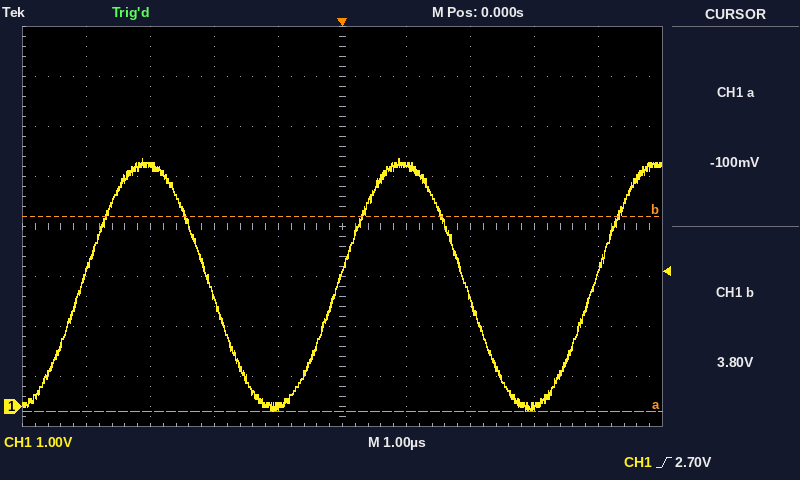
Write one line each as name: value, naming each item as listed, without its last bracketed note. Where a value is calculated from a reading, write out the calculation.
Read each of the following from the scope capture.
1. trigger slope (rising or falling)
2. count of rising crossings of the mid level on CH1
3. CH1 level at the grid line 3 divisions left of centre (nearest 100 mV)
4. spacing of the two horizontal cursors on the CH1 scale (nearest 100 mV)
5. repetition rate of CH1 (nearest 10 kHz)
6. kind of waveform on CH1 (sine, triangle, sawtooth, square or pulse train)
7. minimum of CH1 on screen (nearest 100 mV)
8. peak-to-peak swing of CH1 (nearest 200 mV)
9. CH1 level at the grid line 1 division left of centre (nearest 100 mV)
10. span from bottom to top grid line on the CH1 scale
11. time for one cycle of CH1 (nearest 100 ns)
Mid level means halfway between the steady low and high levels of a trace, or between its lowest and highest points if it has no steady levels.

trigger slope: rising
count of rising crossings of the mid level on CH1: 3
CH1 level at the grid line 3 divisions left of centre: 4.8 V
spacing of the two horizontal cursors on the CH1 scale: 3.9 V
repetition rate of CH1: 1 / 4.0 µs ≈ 250 kHz
kind of waveform on CH1: sine
minimum of CH1 on screen: -100 mV
peak-to-peak swing of CH1: 5.0 V
CH1 level at the grid line 1 division left of centre: 0.0 V
span from bottom to top grid line on the CH1 scale: 8 V
time for one cycle of CH1: 4.0 µs
